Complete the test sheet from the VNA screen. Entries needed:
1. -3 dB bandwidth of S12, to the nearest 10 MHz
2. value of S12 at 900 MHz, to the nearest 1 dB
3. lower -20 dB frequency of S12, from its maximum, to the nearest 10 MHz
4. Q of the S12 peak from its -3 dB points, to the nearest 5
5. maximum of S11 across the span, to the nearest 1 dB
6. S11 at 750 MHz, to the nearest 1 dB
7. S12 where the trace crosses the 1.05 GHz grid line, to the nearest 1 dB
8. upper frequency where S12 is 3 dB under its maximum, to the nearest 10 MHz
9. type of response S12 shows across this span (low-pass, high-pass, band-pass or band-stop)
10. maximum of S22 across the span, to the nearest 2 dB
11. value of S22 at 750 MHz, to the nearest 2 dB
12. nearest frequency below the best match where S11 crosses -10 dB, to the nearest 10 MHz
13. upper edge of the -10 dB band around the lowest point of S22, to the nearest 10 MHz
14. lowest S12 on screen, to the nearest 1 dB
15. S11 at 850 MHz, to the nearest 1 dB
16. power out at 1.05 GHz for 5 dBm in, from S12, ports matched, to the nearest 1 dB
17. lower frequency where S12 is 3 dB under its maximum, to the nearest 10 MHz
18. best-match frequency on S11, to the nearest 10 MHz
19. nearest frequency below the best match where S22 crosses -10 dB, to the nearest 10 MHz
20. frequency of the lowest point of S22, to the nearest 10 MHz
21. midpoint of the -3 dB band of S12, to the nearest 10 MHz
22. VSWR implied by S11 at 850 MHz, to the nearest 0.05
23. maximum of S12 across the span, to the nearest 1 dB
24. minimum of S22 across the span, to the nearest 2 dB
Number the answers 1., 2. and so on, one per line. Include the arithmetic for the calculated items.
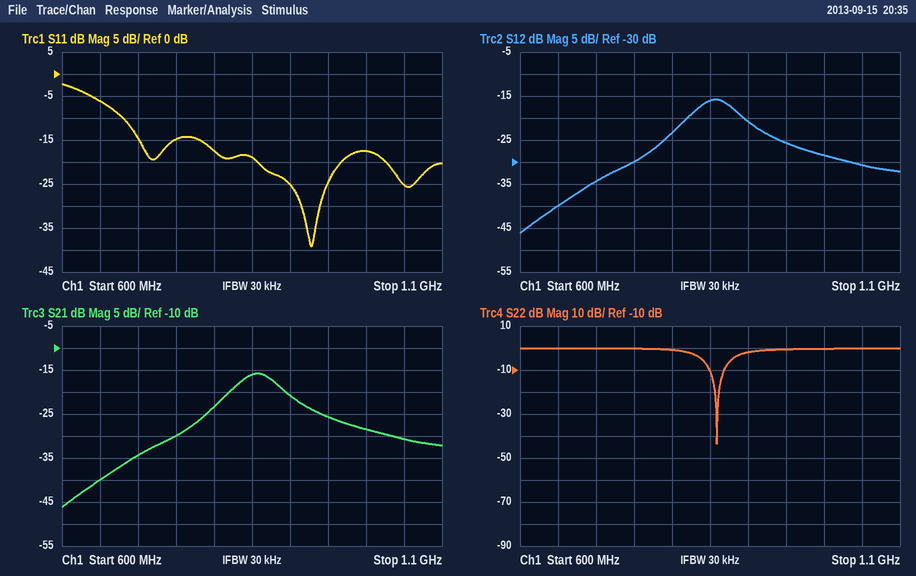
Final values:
1. 890 MHz − 830 MHz = 60 MHz
2. -21 dB
3. 690 MHz
4. 860 MHz / 60 MHz ≈ 14.3, so 15 to the nearest 5
5. -2 dB
6. -15 dB
7. -31 dB
8. 890 MHz
9. band-pass
10. 0 dB
11. 0 dB
12. 680 MHz
13. 870 MHz
14. -46 dB
15. -19 dB
16. 5 dBm + (-31 dB) = -26 dBm
17. 830 MHz
18. 930 MHz
19. 850 MHz
20. 860 MHz
21. 860 MHz
22. |Γ| = 10^(-19/20) = 0.1122; VSWR = (1 + 0.1122)/(1 − 0.1122) ≈ 1.25
23. -16 dB
24. -44 dB
